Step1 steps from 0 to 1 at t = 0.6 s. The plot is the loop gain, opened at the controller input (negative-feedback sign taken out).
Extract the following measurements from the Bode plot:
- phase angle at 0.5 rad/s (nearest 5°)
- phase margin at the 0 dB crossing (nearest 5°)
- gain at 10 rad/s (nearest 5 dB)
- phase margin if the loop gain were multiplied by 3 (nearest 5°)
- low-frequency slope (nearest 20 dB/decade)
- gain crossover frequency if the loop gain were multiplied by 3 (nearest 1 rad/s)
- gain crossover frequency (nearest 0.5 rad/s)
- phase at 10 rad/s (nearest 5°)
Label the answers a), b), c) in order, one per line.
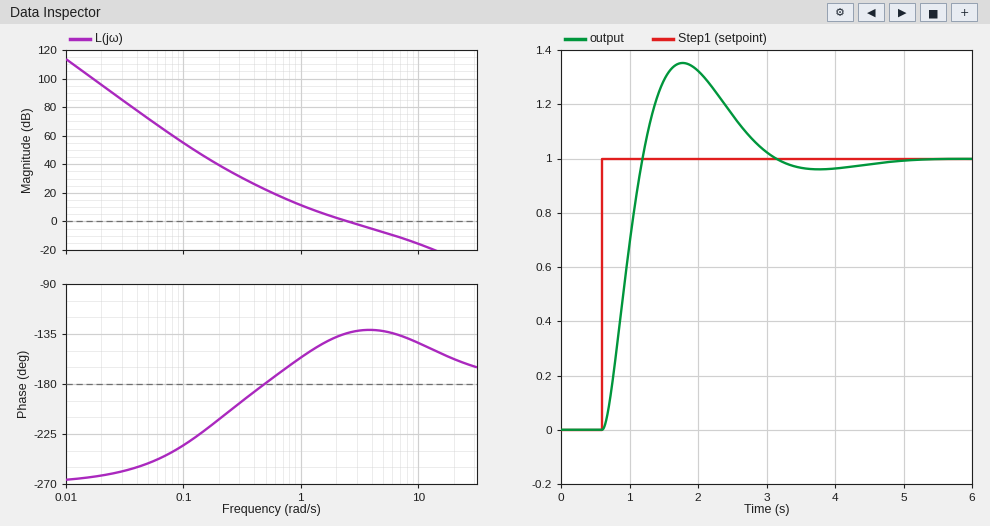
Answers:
a) -180°
b) 45°
c) -15 dB
d) 45°
e) -60 dB/decade
f) 6 rad/s
g) 2.5 rad/s
h) -145°
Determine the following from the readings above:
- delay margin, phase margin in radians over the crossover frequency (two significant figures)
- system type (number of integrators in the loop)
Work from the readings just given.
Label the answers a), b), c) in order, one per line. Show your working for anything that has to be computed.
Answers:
a) 45 × π / 180 / 2.5 = 0.31 s
b) 3
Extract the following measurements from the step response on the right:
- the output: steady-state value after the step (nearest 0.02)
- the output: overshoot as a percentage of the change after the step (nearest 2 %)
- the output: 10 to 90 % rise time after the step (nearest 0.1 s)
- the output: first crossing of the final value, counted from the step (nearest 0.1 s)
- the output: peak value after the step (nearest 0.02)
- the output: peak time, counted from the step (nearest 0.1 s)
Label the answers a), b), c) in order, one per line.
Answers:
a) 1.00
b) 36 %
c) 0.4 s
d) 0.6 s
e) 1.36
f) 1.2 s
